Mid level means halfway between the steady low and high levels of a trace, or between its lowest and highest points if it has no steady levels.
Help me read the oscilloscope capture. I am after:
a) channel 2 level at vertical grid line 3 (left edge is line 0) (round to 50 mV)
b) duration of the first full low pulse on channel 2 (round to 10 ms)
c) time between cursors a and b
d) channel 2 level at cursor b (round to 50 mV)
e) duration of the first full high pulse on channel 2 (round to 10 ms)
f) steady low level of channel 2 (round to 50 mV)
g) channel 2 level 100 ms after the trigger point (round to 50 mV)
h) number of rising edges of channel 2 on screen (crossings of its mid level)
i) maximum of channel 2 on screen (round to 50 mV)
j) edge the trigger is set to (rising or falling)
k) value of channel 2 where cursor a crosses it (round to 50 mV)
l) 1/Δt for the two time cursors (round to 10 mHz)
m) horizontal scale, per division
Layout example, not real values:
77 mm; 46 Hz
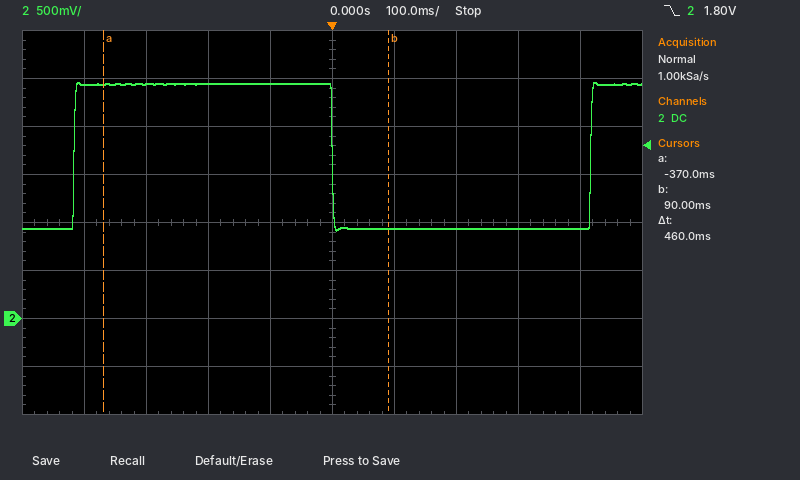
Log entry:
2.45 V; 420 ms; 460 ms; 950 mV; 420 ms; 950 mV; 950 mV; 2; 2.45 V; falling; 2.45 V; 2.17 Hz; 100 ms
